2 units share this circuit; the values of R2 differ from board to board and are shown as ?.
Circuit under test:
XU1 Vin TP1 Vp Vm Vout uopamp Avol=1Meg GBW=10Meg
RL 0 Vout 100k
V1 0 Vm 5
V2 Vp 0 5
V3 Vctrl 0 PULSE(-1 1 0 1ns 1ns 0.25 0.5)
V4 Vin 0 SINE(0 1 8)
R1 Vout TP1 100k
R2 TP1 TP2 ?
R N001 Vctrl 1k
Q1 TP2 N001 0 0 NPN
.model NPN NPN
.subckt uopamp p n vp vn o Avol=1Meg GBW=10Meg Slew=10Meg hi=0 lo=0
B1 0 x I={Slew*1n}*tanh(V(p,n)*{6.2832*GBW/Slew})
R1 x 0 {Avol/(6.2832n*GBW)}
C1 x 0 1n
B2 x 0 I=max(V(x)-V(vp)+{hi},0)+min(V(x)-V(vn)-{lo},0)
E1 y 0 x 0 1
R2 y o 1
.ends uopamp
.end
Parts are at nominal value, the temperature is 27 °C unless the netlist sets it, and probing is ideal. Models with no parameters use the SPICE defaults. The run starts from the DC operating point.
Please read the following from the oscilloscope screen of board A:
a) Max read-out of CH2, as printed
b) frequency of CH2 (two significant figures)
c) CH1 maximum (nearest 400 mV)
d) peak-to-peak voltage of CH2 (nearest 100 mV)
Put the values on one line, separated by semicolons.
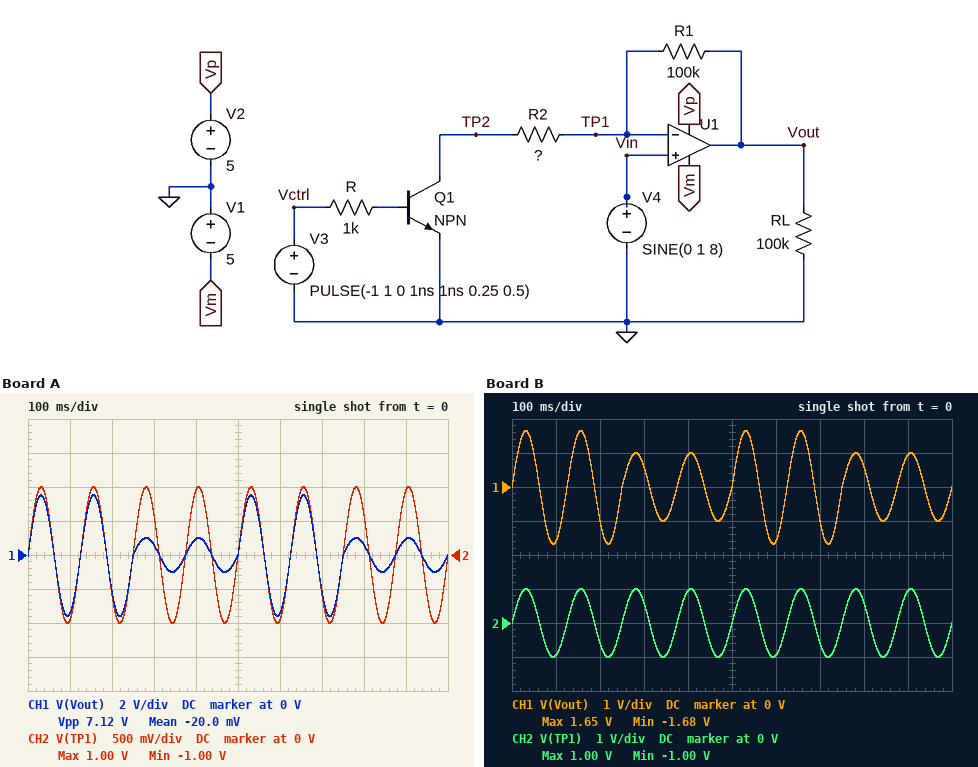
1.00 V; 8.0 Hz; 3.6 V; 2.0 V
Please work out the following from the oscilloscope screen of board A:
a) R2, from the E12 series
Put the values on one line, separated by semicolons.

39 kΩ
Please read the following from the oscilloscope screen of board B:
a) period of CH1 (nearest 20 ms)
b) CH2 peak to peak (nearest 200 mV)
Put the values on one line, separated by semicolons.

120 ms; 2.0 V
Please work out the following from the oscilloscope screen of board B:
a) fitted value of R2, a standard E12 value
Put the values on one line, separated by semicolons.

150 kΩ
